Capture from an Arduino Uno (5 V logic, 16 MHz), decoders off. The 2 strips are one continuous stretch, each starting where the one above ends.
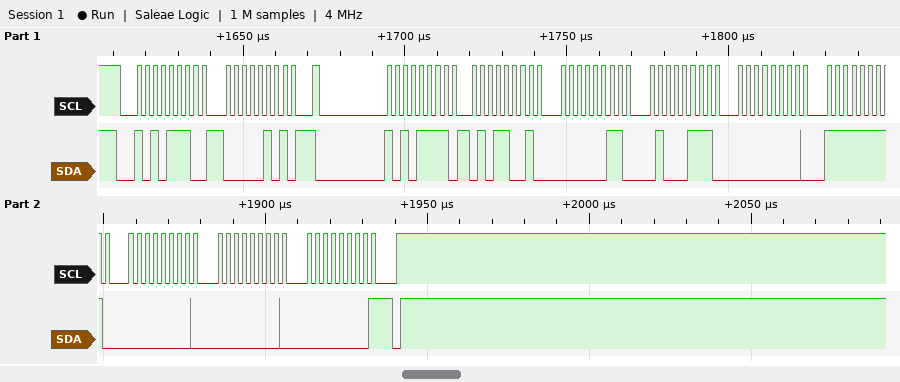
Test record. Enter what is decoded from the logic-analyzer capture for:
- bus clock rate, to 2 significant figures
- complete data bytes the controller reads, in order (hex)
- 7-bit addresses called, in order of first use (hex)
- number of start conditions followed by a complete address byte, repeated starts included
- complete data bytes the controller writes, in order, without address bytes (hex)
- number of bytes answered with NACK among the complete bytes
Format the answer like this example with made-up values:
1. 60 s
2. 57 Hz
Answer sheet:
1. 400 kHz
2. 59 03 47 00 FF 00 00 00
3. 0x57
4. 2
5. 05
6. 1
